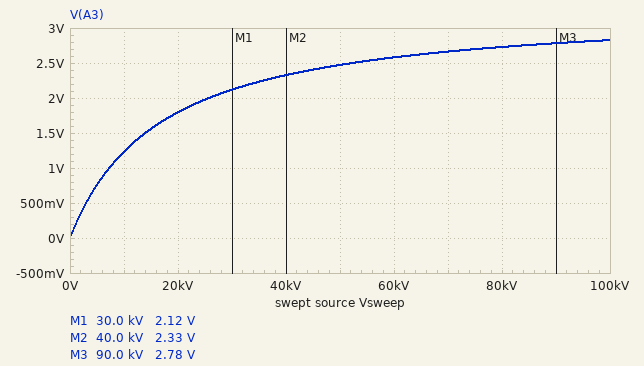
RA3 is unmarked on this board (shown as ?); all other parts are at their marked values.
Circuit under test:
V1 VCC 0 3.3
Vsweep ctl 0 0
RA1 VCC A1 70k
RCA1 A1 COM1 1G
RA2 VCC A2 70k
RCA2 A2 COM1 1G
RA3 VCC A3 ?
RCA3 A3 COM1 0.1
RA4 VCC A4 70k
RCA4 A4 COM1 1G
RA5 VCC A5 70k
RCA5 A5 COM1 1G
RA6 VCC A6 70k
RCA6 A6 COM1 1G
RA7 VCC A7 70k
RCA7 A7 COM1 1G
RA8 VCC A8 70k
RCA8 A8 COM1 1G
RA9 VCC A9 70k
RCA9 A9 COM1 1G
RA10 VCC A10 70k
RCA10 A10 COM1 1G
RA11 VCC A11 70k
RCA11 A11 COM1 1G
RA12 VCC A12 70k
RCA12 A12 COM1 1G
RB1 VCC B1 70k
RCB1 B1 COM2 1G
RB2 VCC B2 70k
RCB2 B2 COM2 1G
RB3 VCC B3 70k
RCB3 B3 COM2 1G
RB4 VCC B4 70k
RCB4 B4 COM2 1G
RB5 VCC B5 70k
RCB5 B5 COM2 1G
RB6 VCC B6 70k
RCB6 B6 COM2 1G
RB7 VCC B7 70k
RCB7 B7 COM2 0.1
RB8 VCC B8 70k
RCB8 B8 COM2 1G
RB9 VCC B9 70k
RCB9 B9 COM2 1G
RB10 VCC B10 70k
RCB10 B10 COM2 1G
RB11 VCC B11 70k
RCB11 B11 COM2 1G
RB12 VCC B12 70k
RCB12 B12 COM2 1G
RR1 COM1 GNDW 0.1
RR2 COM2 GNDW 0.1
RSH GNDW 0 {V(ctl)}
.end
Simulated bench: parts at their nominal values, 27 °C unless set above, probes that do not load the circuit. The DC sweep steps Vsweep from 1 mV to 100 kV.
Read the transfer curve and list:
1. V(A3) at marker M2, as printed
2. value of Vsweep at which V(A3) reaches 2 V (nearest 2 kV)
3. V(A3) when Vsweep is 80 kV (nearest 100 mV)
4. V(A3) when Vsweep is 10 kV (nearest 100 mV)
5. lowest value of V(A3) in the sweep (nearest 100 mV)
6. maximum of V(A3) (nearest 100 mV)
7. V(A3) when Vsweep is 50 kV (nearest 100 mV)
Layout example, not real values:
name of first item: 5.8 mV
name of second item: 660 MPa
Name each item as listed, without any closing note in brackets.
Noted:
V(A3) at marker M2, as printed: 2.33 V
value of Vsweep at which V(A3) reaches 2 V: 26 kV
V(A3) when Vsweep is 80 kV: 2.7 V
V(A3) when Vsweep is 10 kV: 1.2 V
lowest value of V(A3) in the sweep: 0 V
maximum of V(A3): 2.8 V
V(A3) when Vsweep is 50 kV: 2.5 V
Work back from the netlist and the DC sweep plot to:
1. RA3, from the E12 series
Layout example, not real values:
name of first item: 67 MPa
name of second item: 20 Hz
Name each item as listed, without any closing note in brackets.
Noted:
RA3, from the E12 series: 22 kΩ
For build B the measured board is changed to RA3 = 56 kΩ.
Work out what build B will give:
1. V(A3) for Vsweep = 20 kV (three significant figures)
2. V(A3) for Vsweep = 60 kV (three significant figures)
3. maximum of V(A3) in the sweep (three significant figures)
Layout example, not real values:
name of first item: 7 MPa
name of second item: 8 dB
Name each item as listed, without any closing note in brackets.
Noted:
V(A3) for Vsweep = 20 kV: 1.29 V
V(A3) for Vsweep = 60 kV: 2.17 V
maximum of V(A3) in the sweep: 2.52 V
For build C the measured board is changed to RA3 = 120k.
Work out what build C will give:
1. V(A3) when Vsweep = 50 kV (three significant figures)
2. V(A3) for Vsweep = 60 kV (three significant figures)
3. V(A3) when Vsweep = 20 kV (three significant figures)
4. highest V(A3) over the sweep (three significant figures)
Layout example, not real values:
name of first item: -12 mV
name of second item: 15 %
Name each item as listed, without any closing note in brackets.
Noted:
V(A3) when Vsweep = 50 kV: 1.75 V
V(A3) for Vsweep = 60 kV: 1.90 V
V(A3) when Vsweep = 20 kV: 1.03 V
highest V(A3) over the sweep: 2.29 V
